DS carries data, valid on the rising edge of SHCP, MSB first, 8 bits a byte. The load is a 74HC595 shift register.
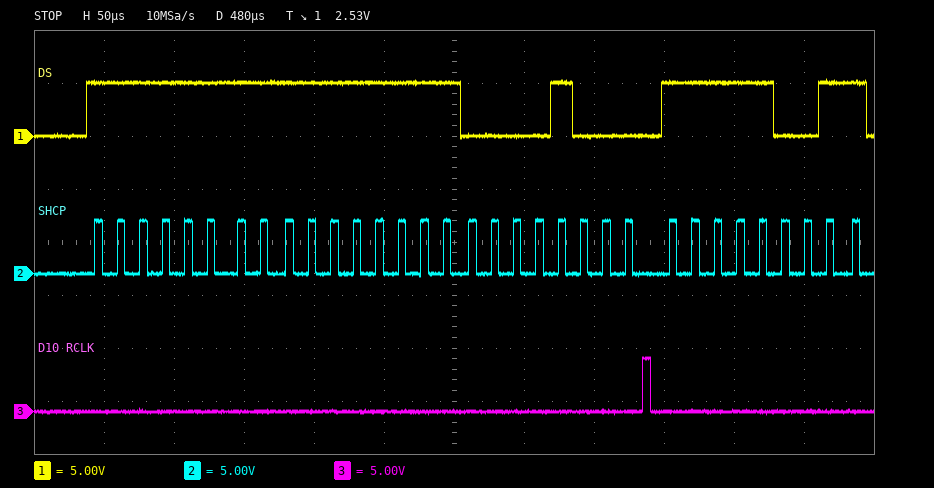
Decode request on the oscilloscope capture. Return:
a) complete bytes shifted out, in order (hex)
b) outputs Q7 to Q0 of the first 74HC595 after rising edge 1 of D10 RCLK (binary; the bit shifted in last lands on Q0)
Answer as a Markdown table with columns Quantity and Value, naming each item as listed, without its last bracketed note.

| Quantity | Value |
|---|---|
| complete bytes shifted out, in order | 0xFF 0xFF 0x08 0xF9 |
| outputs Q7 to Q0 of the first 74HC595 after rising edge 1 of D10 RCLK | 00001000 |
